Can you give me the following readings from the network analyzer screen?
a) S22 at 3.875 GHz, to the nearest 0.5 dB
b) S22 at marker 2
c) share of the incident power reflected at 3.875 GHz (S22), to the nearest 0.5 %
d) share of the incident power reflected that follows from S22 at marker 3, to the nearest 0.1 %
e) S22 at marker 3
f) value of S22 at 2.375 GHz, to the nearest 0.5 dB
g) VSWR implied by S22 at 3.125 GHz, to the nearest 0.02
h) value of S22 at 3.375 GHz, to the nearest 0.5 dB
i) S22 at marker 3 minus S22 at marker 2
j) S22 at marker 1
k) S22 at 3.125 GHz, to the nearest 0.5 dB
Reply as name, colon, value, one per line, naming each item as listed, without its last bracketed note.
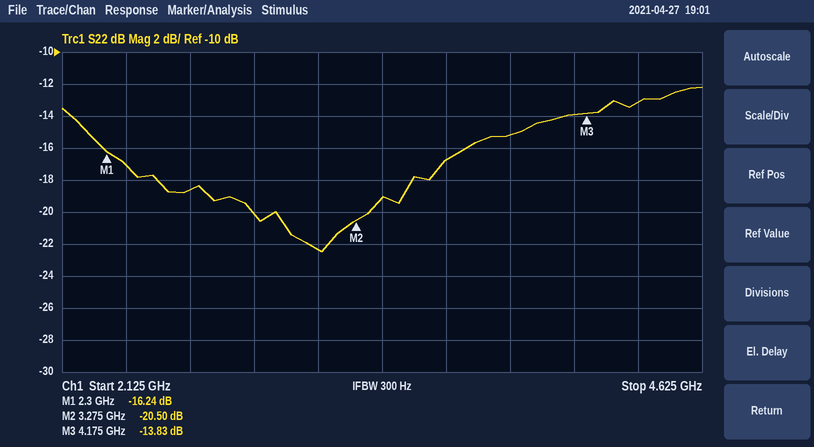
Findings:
S22 at 3.875 GHz, to the nearest 0.5 dB: -15.0 dB
S22 at marker 2: -20.50 dB
share of the incident power reflected at 3.875 GHz (S22), to the nearest 0.5 %: 3.0 %
share of the incident power reflected that follows from S22 at marker 3, to the nearest 0.1 %: 4.1 %
S22 at marker 3: -13.83 dB
value of S22 at 2.375 GHz, to the nearest 0.5 dB: -17.0 dB
VSWR implied by S22 at 3.125 GHz, to the nearest 0.02: 1.16
value of S22 at 3.375 GHz, to the nearest 0.5 dB: -19.0 dB
S22 at marker 3 minus S22 at marker 2: 6.67 dB
S22 at marker 1: -16.24 dB
S22 at 3.125 GHz, to the nearest 0.5 dB: -22.5 dB
